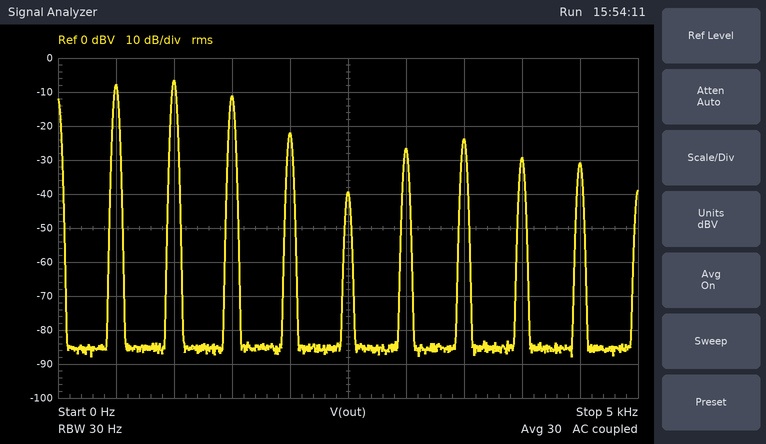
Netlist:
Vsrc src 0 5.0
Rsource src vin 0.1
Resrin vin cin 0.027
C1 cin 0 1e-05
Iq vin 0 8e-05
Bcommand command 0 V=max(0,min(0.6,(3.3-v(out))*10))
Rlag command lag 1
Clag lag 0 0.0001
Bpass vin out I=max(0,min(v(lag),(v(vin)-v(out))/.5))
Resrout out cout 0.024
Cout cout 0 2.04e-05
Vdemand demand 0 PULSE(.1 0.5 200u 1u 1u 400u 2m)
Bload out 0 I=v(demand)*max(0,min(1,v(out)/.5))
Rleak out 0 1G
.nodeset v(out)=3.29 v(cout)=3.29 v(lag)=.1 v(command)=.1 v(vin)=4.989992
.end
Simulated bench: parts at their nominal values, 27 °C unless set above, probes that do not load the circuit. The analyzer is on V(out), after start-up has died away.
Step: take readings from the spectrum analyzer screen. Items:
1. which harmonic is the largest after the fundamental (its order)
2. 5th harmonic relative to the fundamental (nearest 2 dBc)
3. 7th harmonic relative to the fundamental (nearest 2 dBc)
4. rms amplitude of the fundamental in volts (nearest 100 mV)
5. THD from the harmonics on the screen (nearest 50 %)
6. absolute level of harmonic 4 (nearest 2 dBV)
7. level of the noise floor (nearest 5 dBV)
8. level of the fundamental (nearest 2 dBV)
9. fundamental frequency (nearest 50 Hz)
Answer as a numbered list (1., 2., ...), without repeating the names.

1. 2
2. -32 dBc
3. -16 dBc
4. 400 mV
5. 150 %
6. -22 dBV
7. -85 dBV
8. -8 dBV
9. 500 Hz
